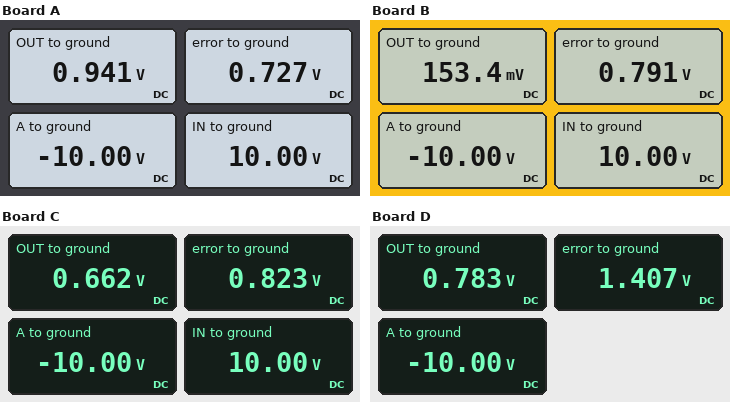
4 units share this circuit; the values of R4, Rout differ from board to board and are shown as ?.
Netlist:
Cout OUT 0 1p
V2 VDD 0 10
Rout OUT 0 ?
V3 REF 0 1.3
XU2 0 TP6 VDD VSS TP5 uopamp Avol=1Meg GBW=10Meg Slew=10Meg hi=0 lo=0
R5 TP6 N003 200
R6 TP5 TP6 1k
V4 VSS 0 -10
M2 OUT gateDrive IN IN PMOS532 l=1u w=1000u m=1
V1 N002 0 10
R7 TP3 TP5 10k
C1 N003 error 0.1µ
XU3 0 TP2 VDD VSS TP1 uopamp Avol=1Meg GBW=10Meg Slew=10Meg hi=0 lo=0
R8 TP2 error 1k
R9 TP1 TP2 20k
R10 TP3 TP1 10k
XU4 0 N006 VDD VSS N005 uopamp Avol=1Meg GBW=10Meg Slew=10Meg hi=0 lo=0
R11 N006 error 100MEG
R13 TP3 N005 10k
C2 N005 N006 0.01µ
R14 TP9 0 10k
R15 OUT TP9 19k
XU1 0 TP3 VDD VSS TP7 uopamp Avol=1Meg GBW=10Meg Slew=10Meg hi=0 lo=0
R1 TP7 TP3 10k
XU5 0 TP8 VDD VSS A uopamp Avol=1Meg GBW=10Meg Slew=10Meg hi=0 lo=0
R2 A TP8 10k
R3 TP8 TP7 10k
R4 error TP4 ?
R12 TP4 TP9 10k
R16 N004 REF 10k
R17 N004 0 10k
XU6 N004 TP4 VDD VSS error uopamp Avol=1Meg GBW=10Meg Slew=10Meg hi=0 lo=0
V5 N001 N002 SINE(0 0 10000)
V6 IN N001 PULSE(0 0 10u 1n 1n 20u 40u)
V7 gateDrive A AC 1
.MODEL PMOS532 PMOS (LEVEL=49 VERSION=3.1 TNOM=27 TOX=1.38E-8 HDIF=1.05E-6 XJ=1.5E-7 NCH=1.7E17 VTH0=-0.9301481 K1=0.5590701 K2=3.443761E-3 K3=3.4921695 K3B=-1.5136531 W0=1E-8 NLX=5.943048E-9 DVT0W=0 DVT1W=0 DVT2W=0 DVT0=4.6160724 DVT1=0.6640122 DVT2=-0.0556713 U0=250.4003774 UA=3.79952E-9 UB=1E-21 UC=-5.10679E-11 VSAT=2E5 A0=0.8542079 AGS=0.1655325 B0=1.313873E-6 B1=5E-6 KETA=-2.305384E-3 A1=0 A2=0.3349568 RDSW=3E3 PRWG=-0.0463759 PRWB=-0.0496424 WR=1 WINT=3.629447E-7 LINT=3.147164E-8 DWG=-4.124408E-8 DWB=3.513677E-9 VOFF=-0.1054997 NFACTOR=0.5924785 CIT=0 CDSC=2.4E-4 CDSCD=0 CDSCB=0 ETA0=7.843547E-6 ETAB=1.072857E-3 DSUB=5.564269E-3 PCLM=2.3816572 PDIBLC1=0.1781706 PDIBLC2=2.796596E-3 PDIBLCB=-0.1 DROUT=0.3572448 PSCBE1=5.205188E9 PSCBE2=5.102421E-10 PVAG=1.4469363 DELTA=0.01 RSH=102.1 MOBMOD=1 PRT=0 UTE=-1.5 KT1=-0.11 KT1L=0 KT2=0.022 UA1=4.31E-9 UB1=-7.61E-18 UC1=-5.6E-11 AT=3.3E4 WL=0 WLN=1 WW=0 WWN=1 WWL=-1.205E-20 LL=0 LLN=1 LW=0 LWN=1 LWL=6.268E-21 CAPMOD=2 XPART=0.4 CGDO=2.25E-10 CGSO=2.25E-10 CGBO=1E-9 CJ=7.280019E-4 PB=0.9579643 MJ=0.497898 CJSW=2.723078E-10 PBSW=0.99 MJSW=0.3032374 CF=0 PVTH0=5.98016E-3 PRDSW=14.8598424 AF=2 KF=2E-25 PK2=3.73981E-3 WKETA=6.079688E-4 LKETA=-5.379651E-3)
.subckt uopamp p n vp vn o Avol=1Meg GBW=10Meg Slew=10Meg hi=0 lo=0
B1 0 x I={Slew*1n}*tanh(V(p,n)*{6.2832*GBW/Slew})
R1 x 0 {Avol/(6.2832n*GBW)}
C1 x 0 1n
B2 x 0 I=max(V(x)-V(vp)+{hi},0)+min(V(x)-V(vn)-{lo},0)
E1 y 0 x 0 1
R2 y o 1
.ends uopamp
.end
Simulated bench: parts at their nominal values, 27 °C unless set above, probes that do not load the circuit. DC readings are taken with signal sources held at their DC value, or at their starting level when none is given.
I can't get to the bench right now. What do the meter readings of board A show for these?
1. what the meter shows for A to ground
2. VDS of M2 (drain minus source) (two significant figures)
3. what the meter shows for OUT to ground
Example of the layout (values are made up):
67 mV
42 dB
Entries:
-10.00 V
-9.1 V
0.941 V
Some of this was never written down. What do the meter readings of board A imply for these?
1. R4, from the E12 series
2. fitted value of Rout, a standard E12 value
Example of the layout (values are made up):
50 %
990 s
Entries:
3.9 kΩ
22 Ω
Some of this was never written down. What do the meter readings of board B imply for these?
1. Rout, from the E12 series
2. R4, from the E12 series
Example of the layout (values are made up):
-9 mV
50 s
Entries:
3.3 Ω
3.9 kΩ
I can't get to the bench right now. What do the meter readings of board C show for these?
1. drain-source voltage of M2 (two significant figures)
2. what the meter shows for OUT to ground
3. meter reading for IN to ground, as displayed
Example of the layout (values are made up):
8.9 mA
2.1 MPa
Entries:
-9.3 V
0.662 V
10.00 V
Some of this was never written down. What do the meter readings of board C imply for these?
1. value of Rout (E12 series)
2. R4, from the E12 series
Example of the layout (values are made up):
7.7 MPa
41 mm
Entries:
15 Ω
6.8 kΩ
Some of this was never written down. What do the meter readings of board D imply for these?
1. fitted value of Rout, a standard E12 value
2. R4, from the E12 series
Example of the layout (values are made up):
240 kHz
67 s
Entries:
18 Ω
33 kΩ
